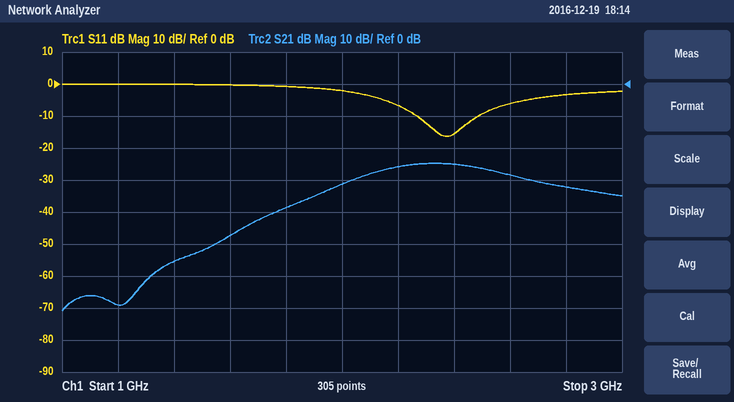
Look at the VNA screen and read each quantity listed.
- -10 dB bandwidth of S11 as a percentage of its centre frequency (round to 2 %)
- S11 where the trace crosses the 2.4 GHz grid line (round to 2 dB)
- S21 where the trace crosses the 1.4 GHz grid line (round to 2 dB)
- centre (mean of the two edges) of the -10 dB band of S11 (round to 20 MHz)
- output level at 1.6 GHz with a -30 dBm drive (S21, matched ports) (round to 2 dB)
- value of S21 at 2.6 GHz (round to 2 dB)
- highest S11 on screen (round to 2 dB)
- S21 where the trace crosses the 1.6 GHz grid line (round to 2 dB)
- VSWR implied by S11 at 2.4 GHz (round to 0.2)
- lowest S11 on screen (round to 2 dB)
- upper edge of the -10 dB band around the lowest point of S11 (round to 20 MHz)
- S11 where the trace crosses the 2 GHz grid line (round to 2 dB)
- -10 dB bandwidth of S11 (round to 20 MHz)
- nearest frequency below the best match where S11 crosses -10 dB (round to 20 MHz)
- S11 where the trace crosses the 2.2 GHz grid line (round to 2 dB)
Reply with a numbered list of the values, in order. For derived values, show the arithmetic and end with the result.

1. 220 MHz / 2.37 GHz ≈ 9.28 %, so 10 % to the nearest 2 %
2. -16 dB
3. -56 dB
4. 2.38 GHz
5. -30 dBm + (-48 dB) = -78 dBm
6. -28 dB
7. 0 dB
8. -48 dB
9. |Γ| = 10^(-16/20) = 0.1585; VSWR = (1 + 0.1585)/(1 − 0.1585) ≈ 1.4
10. -16 dB
11. 2.48 GHz
12. -2 dB
13. 2.48 GHz − 2.26 GHz = 220 MHz
14. 2.26 GHz
15. -6 dB
